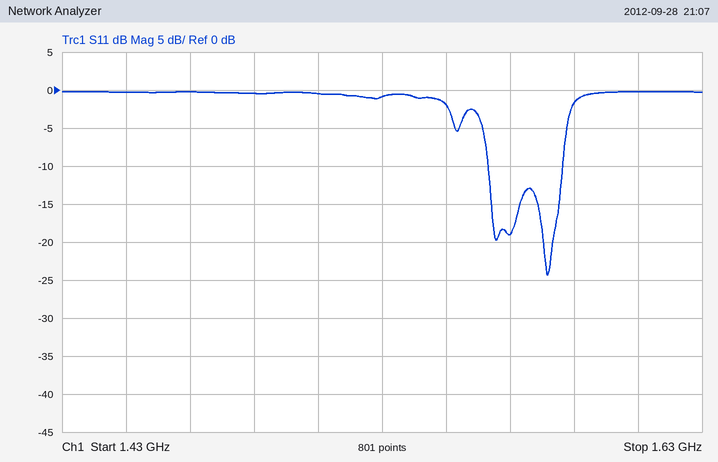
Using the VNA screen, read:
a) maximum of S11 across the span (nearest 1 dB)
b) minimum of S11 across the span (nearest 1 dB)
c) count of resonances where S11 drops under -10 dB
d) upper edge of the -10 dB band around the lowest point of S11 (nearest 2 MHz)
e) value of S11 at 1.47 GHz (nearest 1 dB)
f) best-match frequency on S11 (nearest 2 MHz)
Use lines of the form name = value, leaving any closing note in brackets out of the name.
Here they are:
maximum of S11 across the span = 0 dB
minimum of S11 across the span = -24 dB
count of resonances where S11 drops under -10 dB = 2
upper edge of the -10 dB band around the lowest point of S11 = 1.586 GHz
value of S11 at 1.47 GHz = 0 dB
best-match frequency on S11 = 1.582 GHz
